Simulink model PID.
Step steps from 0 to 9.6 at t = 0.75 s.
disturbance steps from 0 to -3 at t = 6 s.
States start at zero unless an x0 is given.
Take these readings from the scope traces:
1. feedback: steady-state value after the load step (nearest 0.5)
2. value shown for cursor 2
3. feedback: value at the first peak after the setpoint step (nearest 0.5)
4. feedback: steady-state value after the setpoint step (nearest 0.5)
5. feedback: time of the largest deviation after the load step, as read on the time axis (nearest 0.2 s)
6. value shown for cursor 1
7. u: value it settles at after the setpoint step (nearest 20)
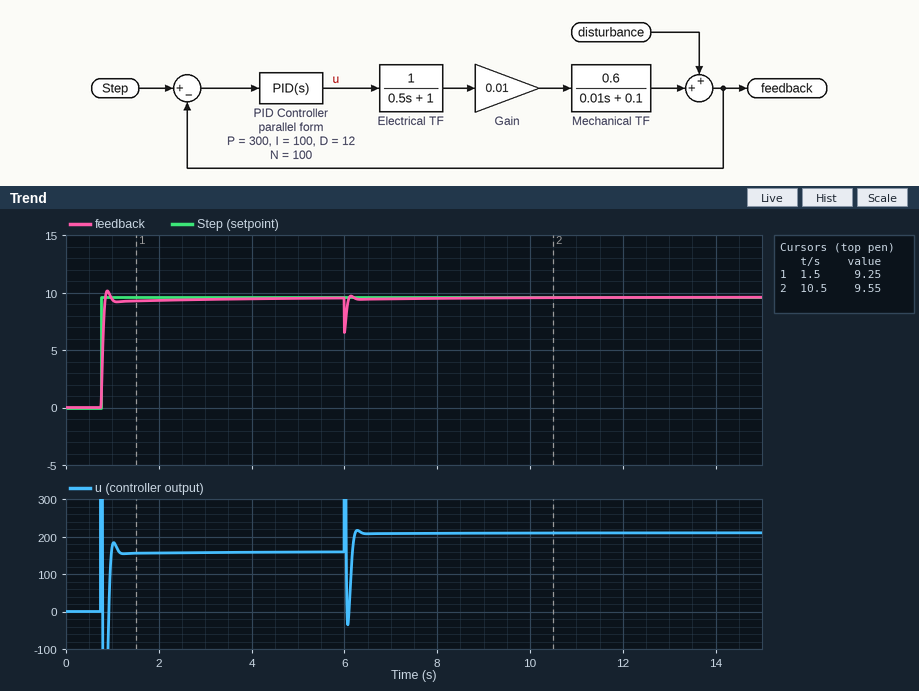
9.5
9.55
10.0
9.5
6.0 s
9.25
160
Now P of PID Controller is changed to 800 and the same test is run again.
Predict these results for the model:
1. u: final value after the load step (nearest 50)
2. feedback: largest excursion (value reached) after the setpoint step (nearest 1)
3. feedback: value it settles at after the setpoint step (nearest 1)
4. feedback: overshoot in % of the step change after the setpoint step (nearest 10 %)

200
12
10
30 %
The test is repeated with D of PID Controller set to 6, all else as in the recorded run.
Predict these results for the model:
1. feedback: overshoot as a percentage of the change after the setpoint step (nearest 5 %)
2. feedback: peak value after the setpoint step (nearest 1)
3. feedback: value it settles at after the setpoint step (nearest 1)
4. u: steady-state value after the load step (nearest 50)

15 %
11
10
200
